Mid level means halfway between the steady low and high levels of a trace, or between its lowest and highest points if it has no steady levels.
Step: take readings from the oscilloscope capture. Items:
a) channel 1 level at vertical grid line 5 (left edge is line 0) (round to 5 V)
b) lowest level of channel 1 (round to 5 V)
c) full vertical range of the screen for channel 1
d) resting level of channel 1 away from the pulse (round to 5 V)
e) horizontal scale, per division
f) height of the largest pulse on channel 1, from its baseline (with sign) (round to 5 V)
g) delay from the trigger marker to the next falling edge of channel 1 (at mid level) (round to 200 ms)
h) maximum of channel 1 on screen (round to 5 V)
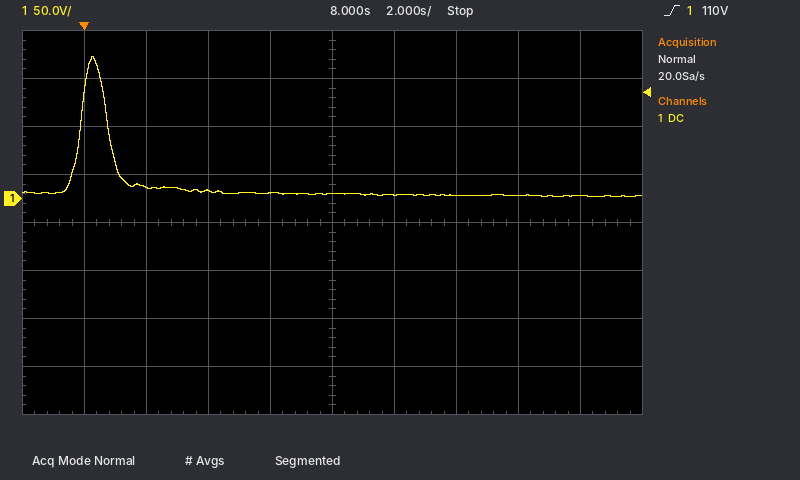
5 V
0 V
400 V
5 V
2 s
+145 V
800 ms
150 V
